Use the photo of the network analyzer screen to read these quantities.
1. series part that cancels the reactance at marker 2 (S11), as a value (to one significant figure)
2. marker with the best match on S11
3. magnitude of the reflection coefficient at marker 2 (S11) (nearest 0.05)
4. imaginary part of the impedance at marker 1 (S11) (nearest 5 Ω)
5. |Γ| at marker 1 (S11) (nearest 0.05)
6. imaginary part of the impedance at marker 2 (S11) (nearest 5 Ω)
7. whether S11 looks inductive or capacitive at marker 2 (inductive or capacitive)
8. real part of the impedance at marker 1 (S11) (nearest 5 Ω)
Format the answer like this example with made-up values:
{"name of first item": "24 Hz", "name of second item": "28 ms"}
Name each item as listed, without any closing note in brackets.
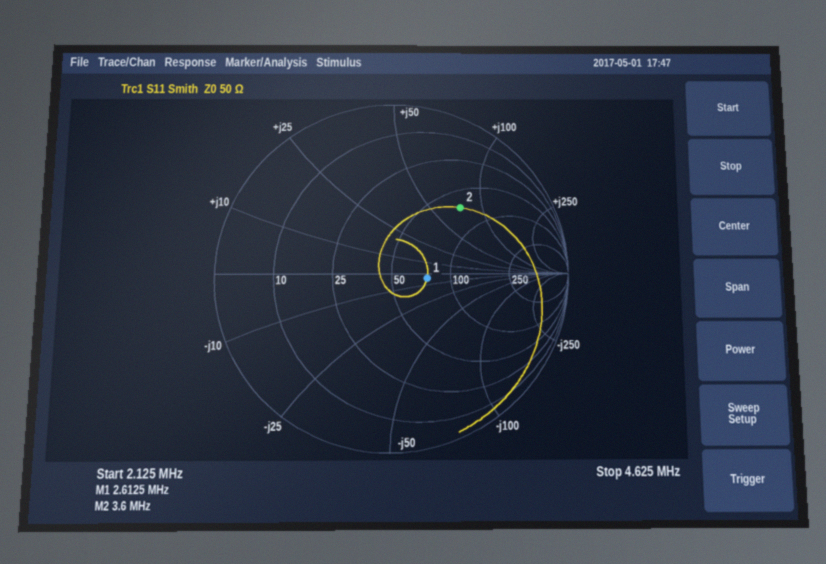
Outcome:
{"series part that cancels the reactance at marker 2 (S11), as a value": "600 pF", "marker with the best match on S11": "marker 1", "magnitude of the reflection coefficient at marker 2 (S11)": "0.55", "imaginary part of the impedance at marker 1 (S11)": "-5 Ω", "|Γ| at marker 1 (S11)": "0.20", "imaginary part of the impedance at marker 2 (S11)": "+75 Ω", "whether S11 looks inductive or capacitive at marker 2": "inductive", "real part of the impedance at marker 1 (S11)": "75 Ω"}
